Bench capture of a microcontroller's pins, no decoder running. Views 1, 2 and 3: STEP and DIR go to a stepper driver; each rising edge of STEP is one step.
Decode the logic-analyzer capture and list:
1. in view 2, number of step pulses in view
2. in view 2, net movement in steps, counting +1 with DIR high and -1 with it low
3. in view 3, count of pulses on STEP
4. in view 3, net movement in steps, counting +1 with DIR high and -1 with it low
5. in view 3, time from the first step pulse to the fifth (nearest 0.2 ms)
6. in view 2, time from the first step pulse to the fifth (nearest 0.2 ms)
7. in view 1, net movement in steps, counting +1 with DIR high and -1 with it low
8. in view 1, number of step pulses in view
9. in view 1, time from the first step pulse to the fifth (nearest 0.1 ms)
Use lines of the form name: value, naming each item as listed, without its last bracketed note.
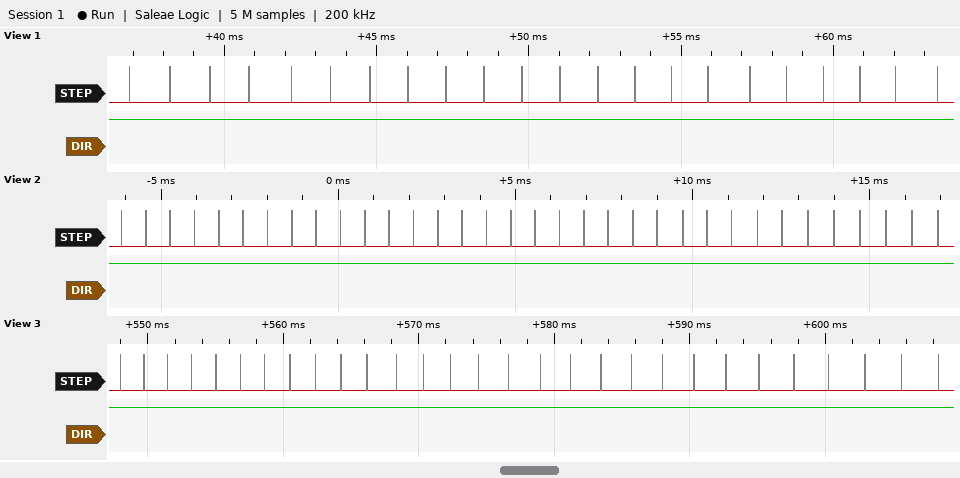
in view 2, number of step pulses in view: 34
in view 2, net movement in steps, counting +1 with DIR high and -1 with it low: +34
in view 3, count of pulses on STEP: 29
in view 3, net movement in steps, counting +1 with DIR high and -1 with it low: +29
in view 3, time from the first step pulse to the fifth: 7.0 ms
in view 2, time from the first step pulse to the fifth: 2.8 ms
in view 1, net movement in steps, counting +1 with DIR high and -1 with it low: +22
in view 1, number of step pulses in view: 22
in view 1, time from the first step pulse to the fifth: 5.3 ms
